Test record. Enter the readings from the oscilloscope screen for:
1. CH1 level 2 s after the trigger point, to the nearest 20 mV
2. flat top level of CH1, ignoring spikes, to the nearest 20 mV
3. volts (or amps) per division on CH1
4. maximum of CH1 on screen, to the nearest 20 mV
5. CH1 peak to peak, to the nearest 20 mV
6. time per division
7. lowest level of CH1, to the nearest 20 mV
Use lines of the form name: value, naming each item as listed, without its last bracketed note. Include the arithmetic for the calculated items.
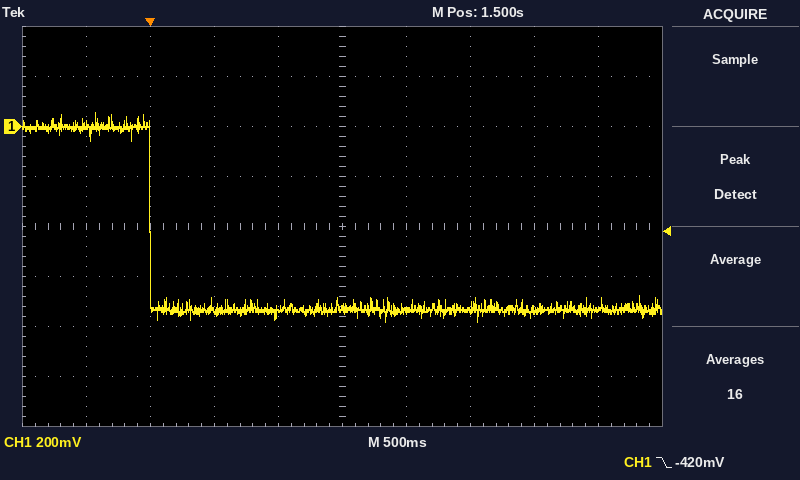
CH1 level 2 s after the trigger point, to the nearest 20 mV: -740 mV
flat top level of CH1, ignoring spikes, to the nearest 20 mV: 0 mV
volts (or amps) per division on CH1: 200 mV
maximum of CH1 on screen, to the nearest 20 mV: 60 mV
CH1 peak to peak, to the nearest 20 mV: 60 mV − (-780 mV) = 840 mV
time per division: 500 ms
lowest level of CH1, to the nearest 20 mV: -780 mV
